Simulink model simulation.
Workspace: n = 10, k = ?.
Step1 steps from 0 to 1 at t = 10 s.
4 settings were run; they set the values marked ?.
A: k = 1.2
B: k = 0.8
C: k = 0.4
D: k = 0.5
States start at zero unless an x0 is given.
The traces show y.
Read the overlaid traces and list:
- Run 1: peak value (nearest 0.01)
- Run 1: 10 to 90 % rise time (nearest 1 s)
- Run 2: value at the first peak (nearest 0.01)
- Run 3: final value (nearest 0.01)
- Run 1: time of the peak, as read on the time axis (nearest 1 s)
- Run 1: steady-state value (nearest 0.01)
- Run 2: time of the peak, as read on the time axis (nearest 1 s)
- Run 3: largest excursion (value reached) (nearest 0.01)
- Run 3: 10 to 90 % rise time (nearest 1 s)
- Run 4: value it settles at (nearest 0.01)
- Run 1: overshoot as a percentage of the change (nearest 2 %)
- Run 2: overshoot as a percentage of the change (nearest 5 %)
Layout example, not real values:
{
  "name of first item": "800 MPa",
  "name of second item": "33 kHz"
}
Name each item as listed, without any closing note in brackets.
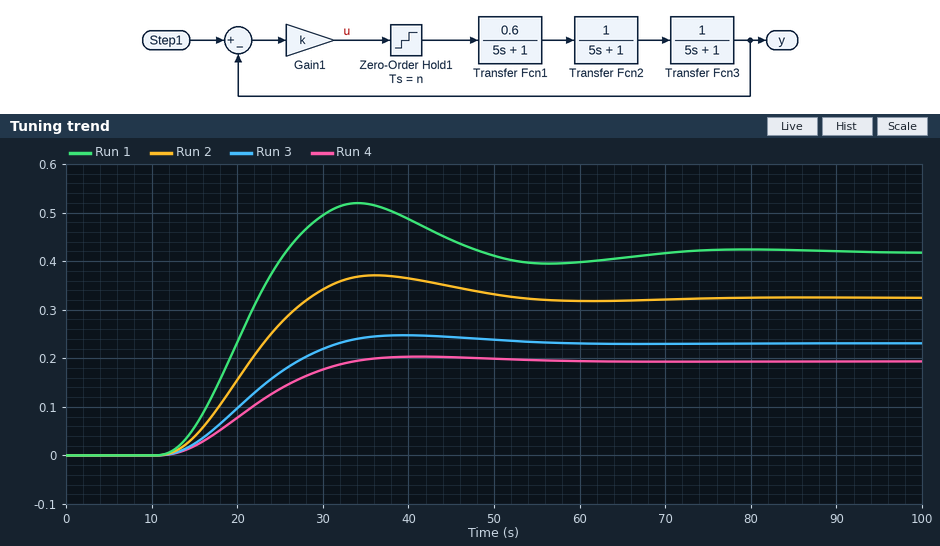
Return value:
{
  "Run 1: peak value": "0.52",
  "Run 1: 10 to 90 % rise time": "10 s",
  "Run 2: value at the first peak": "0.37",
  "Run 3: final value": "0.23",
  "Run 1: time of the peak, as read on the time axis": "34 s",
  "Run 1: steady-state value": "0.42",
  "Run 2: time of the peak, as read on the time axis": "36 s",
  "Run 3: largest excursion (value reached)": "0.25",
  "Run 3: 10 to 90 % rise time": "14 s",
  "Run 4: value it settles at": "0.19",
  "Run 1: overshoot as a percentage of the change": "24 %",
  "Run 2: overshoot as a percentage of the change": "15 %"
}
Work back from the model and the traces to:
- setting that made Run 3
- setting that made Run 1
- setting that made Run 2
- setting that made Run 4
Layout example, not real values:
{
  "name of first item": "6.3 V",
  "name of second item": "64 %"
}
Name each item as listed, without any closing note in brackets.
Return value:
{
  "setting that made Run 3": "D",
  "setting that made Run 1": "A",
  "setting that made Run 2": "B",
  "setting that made Run 4": "C"
}
